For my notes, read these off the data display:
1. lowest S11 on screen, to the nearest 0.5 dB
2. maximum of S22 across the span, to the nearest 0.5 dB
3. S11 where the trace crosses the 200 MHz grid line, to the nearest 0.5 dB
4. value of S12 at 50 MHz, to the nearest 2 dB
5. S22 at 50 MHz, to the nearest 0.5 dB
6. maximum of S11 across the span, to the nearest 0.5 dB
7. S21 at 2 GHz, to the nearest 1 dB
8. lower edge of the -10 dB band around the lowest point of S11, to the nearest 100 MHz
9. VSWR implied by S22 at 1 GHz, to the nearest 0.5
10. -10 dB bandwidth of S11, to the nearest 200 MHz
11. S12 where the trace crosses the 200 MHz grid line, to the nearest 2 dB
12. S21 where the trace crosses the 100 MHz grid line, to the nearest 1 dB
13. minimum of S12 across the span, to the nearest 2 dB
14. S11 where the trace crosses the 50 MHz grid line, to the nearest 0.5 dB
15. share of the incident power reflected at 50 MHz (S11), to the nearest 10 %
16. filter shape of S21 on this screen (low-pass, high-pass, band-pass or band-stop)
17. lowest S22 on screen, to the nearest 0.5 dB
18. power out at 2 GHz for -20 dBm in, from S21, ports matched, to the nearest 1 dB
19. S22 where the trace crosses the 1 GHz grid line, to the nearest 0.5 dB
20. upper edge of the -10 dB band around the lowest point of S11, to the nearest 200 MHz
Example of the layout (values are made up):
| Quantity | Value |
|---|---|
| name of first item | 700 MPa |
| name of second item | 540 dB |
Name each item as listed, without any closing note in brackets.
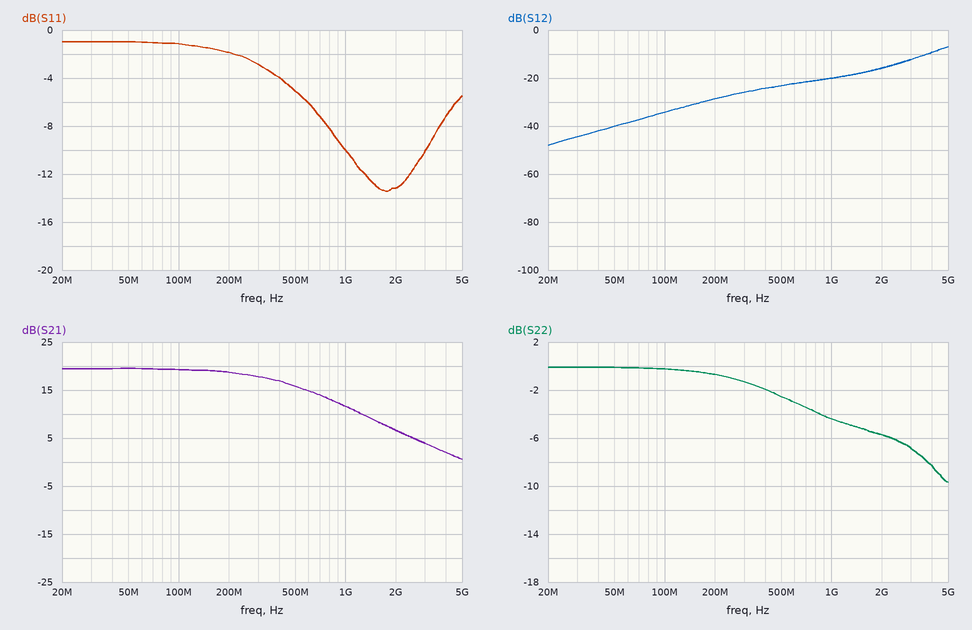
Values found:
| Quantity | Value |
|---|---|
| lowest S11 on screen, to the nearest 0.5 dB | -13.5 dB |
| maximum of S22 across the span, to the nearest 0.5 dB | 0.0 dB |
| S11 where the trace crosses the 200 MHz grid line, to the nearest 0.5 dB | -2.0 dB |
| value of S12 at 50 MHz, to the nearest 2 dB | -40 dB |
| S22 at 50 MHz, to the nearest 0.5 dB | 0.0 dB |
| maximum of S11 across the span, to the nearest 0.5 dB | -1.0 dB |
| S21 at 2 GHz, to the nearest 1 dB | 7 dB |
| lower edge of the -10 dB band around the lowest point of S11, to the nearest 100 MHz | 1.0 GHz |
| VSWR implied by S22 at 1 GHz, to the nearest 0.5 | 4.0 |
| -10 dB bandwidth of S11, to the nearest 200 MHz | 2.0 GHz |
| S12 where the trace crosses the 200 MHz grid line, to the nearest 2 dB | -28 dB |
| S21 where the trace crosses the 100 MHz grid line, to the nearest 1 dB | 19 dB |
| minimum of S12 across the span, to the nearest 2 dB | -48 dB |
| S11 where the trace crosses the 50 MHz grid line, to the nearest 0.5 dB | -1.0 dB |
| share of the incident power reflected at 50 MHz (S11), to the nearest 10 % | 80 % |
| filter shape of S21 on this screen | low-pass |
| lowest S22 on screen, to the nearest 0.5 dB | -9.5 dB |
| power out at 2 GHz for -20 dBm in, from S21, ports matched, to the nearest 1 dB | -13 dBm |
| S22 where the trace crosses the 1 GHz grid line, to the nearest 0.5 dB | -4.5 dB |
| upper edge of the -10 dB band around the lowest point of S11, to the nearest 200 MHz | 3.0 GHz |
